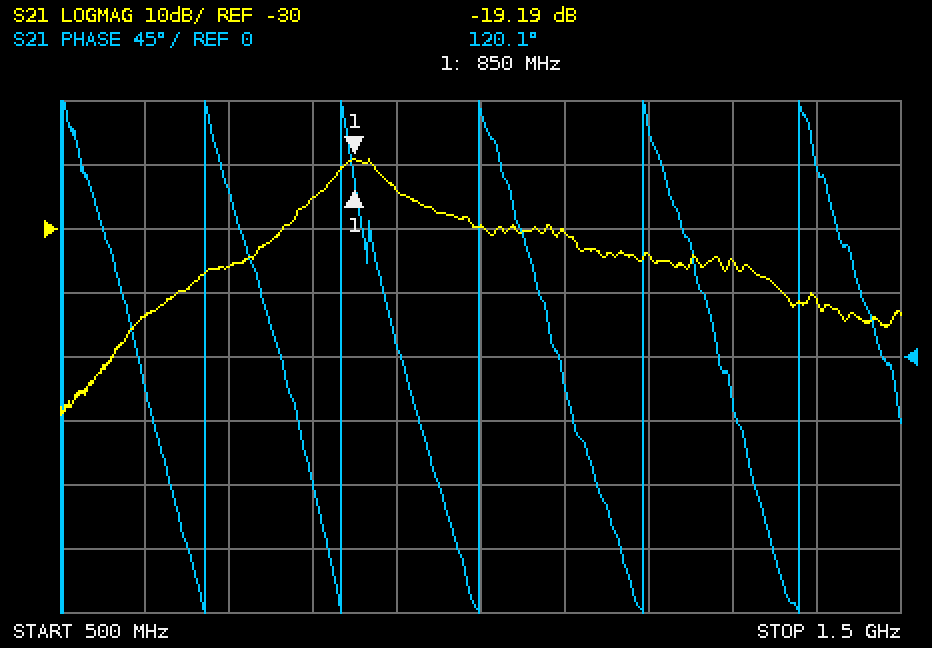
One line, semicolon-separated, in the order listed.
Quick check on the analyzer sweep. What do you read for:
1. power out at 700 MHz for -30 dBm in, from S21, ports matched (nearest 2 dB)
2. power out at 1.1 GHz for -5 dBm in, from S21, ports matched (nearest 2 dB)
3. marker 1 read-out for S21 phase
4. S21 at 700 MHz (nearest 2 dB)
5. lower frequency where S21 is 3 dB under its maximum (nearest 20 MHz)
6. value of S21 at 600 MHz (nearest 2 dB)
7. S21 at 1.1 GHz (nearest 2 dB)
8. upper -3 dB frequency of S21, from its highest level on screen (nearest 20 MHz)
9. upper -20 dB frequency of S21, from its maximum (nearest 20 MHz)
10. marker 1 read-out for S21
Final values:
-66 dBm; -36 dBm; 120.1°; -36 dB; 820 MHz; -44 dB; -30 dB; 880 MHz; 1.36 GHz; -19.19 dB
